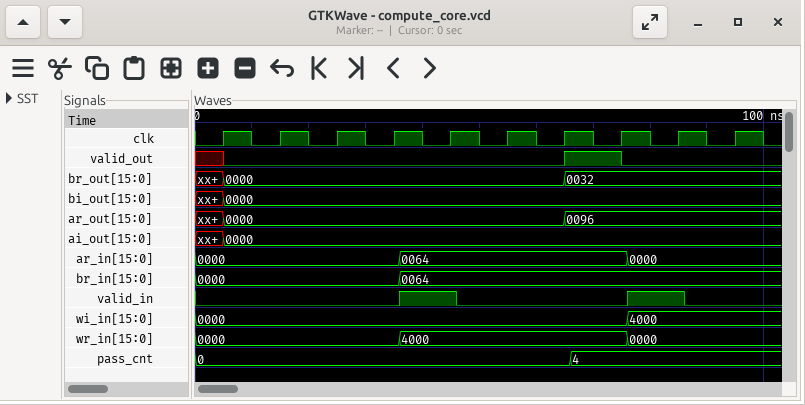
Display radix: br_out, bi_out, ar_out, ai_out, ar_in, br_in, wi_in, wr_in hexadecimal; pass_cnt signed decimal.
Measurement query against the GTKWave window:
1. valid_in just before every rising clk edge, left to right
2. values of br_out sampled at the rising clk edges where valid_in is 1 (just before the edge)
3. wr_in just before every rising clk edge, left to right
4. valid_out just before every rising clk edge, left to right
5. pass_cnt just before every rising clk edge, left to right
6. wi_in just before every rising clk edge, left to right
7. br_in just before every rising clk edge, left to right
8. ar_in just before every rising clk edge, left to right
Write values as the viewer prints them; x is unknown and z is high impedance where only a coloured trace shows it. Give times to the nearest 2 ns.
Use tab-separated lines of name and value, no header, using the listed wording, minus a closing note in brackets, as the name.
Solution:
valid_in just before every rising clk edge, left to right	0 0 0 0 1 0 0 0 1 0
values of br_out sampled at the rising clk edges where valid_in is 1	0000, 0032
wr_in just before every rising clk edge, left to right	0000, 0000, 0000, 0000, 4000, 4000, 4000, 4000, 0000, 0000
valid_out just before every rising clk edge, left to right	x 0 0 0 0 0 0 1 0 0
pass_cnt just before every rising clk edge, left to right	0, 0, 0, 0, 0, 0, 0, 4, 4, 4
wi_in just before every rising clk edge, left to right	0000, 0000, 0000, 0000, 0000, 0000, 0000, 0000, 4000, 4000
br_in just before every rising clk edge, left to right	0000, 0000, 0000, 0000, 0064, 0064, 0064, 0064, 0064, 0064
ar_in just before every rising clk edge, left to right	0000, 0000, 0000, 0000, 0064, 0064, 0064, 0064, 0000, 0000
